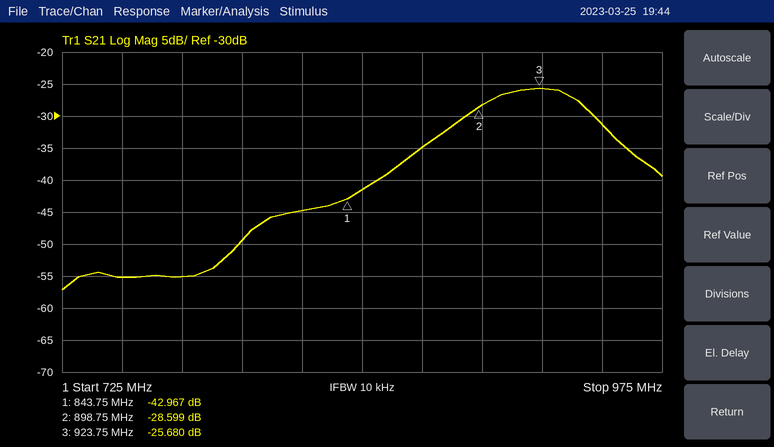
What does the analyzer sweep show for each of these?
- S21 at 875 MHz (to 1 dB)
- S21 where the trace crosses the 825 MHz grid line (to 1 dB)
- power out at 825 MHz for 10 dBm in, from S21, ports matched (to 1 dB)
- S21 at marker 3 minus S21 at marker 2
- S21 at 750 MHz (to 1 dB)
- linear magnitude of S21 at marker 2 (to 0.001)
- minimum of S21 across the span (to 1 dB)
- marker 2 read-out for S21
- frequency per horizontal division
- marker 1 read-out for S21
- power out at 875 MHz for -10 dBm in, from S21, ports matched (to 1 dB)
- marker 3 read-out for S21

-35 dB
-45 dB
-35 dBm
2.919 dB
-55 dB
0.037
-57 dB
-28.599 dB
25 MHz
-42.967 dB
-45 dBm
-25.680 dB
